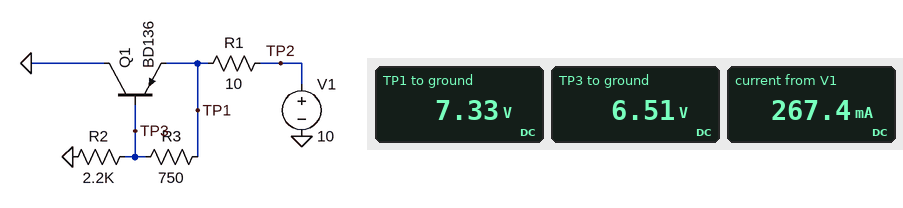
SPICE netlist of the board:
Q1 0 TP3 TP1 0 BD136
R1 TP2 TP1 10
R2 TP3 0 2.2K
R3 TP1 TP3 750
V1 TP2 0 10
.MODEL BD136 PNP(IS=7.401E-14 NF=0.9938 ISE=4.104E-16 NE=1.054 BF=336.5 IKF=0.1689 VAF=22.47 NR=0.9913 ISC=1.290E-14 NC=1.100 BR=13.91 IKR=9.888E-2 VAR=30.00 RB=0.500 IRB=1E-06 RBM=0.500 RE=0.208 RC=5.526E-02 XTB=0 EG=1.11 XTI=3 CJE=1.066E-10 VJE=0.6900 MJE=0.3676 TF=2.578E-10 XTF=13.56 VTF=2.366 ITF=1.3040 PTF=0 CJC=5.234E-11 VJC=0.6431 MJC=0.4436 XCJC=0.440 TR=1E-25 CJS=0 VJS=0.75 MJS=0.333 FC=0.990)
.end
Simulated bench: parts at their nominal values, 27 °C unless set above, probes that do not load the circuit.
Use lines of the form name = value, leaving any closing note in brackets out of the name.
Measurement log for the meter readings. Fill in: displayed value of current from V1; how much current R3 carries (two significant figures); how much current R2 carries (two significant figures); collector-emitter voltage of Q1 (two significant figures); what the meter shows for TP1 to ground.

displayed value of current from V1 = 267.4 mA
how much current R3 carries = 1.1 mA
how much current R2 carries = 3.0 mA
collector-emitter voltage of Q1 = -7.3 V
what the meter shows for TP1 to ground = 7.33 V
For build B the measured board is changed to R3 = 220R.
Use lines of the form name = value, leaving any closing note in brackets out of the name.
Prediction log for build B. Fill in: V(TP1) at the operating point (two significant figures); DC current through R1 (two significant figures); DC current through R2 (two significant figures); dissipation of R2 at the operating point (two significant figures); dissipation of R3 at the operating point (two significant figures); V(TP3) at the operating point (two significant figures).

V(TP1) at the operating point = 9.0 V
DC current through R1 = 98 mA
DC current through R2 = 3.8 mA
dissipation of R2 at the operating point = 31 mW
dissipation of R3 at the operating point = 2.5 mW
V(TP3) at the operating point = 8.3 V
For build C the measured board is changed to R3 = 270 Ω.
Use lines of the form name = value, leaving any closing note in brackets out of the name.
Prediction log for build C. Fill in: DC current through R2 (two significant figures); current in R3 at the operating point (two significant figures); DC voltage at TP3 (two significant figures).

DC current through R2 = 3.5 mA
current in R3 at the operating point = 2.8 mA
DC voltage at TP3 = 7.8 V
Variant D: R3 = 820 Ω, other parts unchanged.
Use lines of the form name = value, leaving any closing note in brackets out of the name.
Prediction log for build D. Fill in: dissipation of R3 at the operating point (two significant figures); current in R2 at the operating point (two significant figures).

dissipation of R3 at the operating point = 810 µW
current in R2 at the operating point = 2.9 mA
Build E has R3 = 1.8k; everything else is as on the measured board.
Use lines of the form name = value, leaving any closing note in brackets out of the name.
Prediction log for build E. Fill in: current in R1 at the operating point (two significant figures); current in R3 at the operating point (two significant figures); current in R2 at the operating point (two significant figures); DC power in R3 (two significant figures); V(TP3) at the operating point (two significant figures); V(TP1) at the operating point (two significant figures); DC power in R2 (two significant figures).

current in R1 at the operating point = 300 mA
current in R3 at the operating point = 460 µA
current in R2 at the operating point = 2.8 mA
DC power in R3 = 380 µW
V(TP3) at the operating point = 6.1 V
V(TP1) at the operating point = 7.0 V
DC power in R2 = 17 mW
